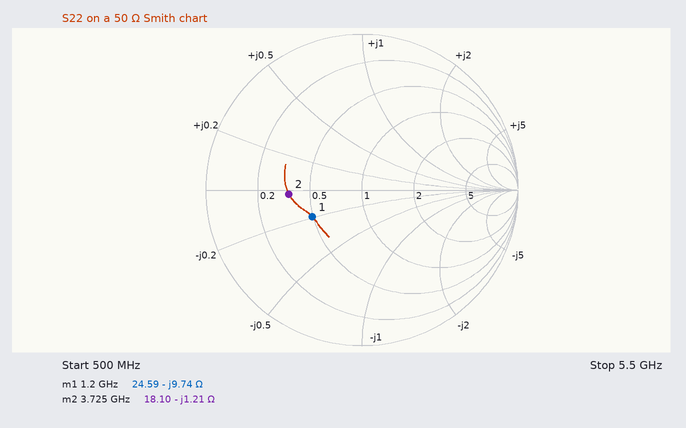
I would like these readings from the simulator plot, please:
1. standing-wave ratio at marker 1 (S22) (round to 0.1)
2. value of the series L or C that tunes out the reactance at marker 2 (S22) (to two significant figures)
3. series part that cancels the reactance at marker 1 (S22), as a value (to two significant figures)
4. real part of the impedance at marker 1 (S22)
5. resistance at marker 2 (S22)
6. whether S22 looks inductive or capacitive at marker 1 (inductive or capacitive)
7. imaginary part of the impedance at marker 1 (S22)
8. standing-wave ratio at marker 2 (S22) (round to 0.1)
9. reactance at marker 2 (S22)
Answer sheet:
2.1
52 pH
1.3 nH
24.59 Ω
18.10 Ω
capacitive
-9.74 Ω
2.8
-1.21 Ω
